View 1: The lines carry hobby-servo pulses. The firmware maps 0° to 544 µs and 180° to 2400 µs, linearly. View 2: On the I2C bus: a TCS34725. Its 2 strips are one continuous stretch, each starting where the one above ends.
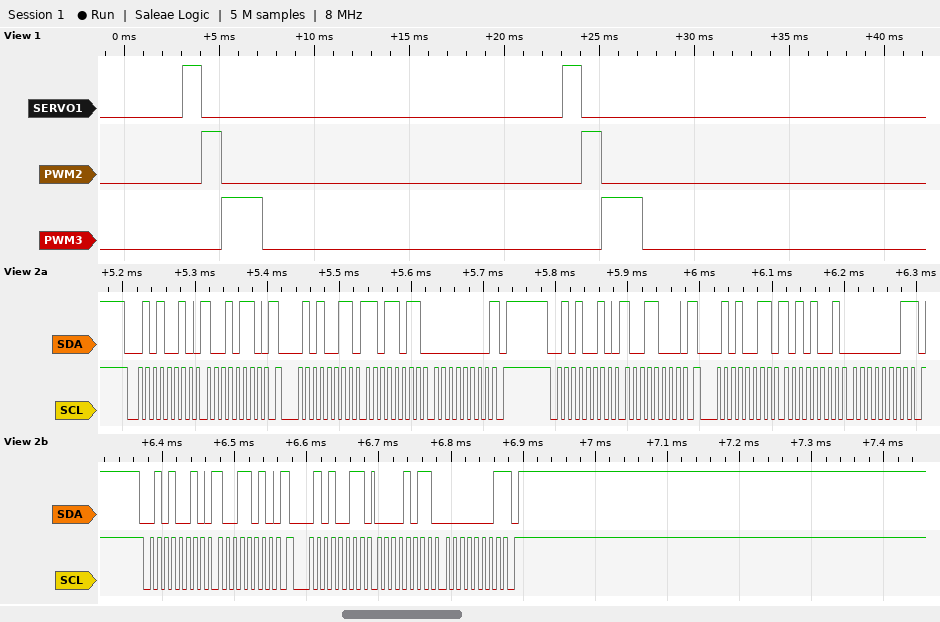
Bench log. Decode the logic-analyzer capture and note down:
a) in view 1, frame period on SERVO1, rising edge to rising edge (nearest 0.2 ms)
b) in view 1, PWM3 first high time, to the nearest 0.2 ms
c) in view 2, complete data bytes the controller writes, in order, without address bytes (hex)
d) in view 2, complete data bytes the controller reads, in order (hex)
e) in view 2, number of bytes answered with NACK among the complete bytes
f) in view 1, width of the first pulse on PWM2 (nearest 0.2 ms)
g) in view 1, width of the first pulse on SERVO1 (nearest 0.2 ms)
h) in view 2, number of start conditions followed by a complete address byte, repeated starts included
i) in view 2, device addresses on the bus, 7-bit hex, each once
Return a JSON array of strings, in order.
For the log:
["20.0 ms", "2.2 ms", "96 98 9A", "DB 00 A9 01 0B 01", "3", "1.0 ms", "1.0 ms", "6", "0x29"]
